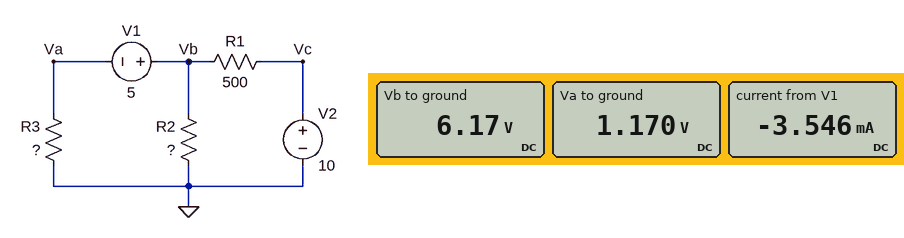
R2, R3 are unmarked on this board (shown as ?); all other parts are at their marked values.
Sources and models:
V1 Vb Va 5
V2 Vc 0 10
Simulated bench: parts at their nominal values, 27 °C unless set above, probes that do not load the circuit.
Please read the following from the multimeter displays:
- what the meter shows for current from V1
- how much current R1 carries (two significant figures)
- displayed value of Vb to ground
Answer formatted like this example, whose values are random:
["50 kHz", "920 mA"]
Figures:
["-3.546 mA", "7.7 mA", "6.17 V"]
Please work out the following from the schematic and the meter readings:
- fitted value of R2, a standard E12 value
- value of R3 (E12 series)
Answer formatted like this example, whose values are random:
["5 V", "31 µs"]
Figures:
["1.5 kΩ", "330 Ω"]
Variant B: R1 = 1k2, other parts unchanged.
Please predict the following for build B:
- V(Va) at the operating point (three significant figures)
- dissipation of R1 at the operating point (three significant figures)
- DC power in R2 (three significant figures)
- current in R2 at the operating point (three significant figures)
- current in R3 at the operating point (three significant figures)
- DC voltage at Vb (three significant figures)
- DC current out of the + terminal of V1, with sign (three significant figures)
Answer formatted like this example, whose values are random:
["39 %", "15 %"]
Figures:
["184 mV", "19.3 mW", "17.9 mW", "3.46 mA", "557 µA", "5.18 V", "-557 µA"]
